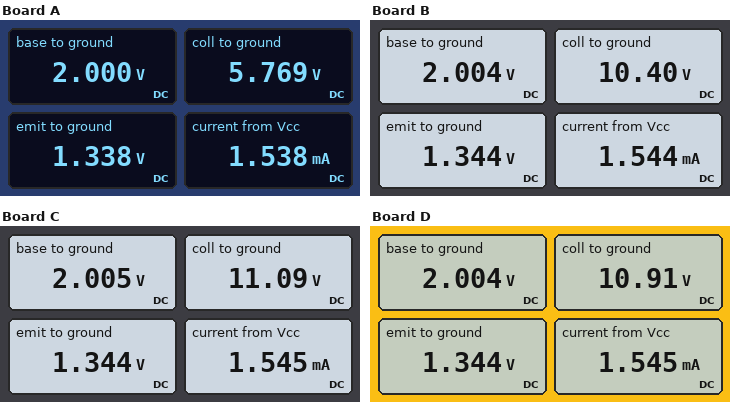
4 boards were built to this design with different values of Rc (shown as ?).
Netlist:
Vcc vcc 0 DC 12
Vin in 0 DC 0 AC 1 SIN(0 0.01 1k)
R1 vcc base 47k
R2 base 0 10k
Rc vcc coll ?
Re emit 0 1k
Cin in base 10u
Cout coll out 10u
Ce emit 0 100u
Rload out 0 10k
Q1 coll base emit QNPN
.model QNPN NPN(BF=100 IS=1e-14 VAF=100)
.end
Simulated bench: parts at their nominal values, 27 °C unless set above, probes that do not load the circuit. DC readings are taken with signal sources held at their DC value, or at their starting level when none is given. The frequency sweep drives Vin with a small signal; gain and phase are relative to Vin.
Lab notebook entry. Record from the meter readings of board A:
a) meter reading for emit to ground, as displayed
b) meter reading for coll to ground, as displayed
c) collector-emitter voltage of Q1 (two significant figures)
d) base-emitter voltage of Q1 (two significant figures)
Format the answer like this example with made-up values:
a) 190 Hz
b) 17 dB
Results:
a) 1.338 V
b) 5.769 V
c) 4.4 V
d) 660 mV
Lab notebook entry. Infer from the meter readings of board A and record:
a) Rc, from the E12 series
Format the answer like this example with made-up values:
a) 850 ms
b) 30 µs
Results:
a) 4.7 kΩ
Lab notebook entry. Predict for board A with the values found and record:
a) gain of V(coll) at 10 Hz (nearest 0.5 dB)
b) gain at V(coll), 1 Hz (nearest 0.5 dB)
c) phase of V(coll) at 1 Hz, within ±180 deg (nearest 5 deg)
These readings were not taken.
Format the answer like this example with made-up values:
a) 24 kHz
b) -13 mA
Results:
a) 25.0 dB
b) 6.0 dB
c) -95 deg
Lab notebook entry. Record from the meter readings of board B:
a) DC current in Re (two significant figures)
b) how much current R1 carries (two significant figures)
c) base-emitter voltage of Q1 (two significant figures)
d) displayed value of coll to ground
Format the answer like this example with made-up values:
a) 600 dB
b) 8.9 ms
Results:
a) 1.3 mA
b) 210 µA
c) 660 mV
d) 10.40 V
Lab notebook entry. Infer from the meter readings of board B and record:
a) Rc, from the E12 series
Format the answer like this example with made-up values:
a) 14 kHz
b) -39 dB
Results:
a) 1.2 kΩ
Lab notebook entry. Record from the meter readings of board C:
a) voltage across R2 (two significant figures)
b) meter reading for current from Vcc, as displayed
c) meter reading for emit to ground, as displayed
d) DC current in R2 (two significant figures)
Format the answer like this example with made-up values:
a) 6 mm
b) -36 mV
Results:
a) 2.0 V
b) 1.545 mA
c) 1.344 V
d) 200 µA
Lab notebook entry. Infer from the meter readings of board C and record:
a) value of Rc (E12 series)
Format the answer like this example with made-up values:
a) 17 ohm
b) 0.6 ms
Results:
a) 680 Ω
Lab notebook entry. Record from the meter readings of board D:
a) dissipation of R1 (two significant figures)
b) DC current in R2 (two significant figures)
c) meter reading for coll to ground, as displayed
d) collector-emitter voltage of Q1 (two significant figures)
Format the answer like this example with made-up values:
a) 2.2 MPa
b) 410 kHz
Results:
a) 2.1 mW
b) 200 µA
c) 10.91 V
d) 9.6 V
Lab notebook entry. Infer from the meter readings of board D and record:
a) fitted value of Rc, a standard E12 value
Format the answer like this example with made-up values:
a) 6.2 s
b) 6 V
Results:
a) 820 Ω
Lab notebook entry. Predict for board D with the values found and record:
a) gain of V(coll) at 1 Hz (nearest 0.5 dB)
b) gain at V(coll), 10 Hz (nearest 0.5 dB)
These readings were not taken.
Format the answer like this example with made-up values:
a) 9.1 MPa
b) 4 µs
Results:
a) -8.0 dB
b) 12.5 dB
